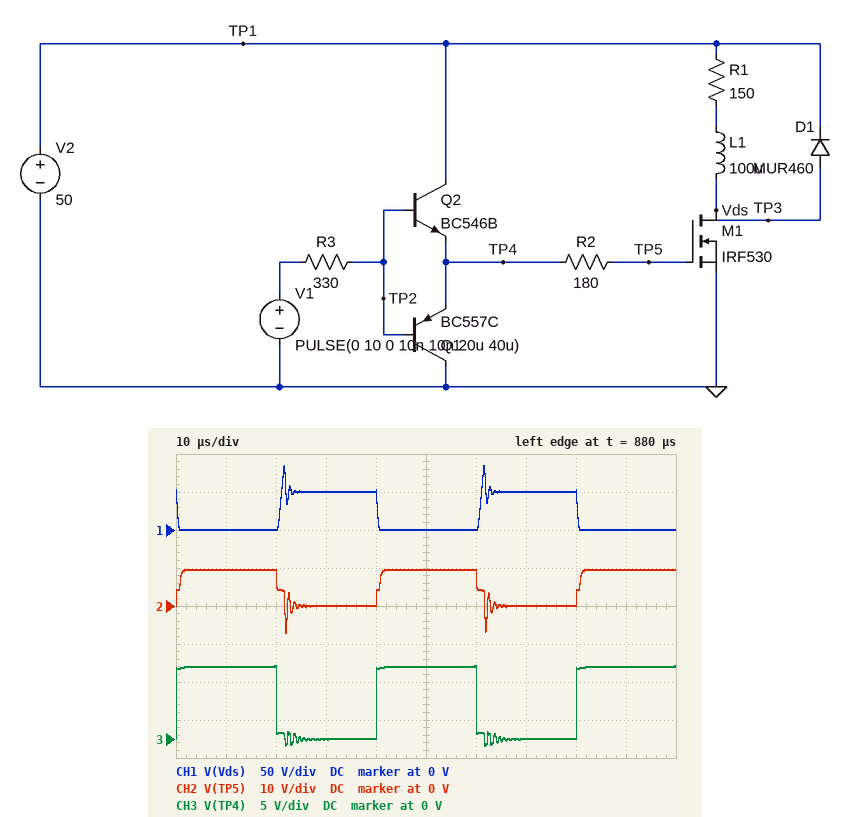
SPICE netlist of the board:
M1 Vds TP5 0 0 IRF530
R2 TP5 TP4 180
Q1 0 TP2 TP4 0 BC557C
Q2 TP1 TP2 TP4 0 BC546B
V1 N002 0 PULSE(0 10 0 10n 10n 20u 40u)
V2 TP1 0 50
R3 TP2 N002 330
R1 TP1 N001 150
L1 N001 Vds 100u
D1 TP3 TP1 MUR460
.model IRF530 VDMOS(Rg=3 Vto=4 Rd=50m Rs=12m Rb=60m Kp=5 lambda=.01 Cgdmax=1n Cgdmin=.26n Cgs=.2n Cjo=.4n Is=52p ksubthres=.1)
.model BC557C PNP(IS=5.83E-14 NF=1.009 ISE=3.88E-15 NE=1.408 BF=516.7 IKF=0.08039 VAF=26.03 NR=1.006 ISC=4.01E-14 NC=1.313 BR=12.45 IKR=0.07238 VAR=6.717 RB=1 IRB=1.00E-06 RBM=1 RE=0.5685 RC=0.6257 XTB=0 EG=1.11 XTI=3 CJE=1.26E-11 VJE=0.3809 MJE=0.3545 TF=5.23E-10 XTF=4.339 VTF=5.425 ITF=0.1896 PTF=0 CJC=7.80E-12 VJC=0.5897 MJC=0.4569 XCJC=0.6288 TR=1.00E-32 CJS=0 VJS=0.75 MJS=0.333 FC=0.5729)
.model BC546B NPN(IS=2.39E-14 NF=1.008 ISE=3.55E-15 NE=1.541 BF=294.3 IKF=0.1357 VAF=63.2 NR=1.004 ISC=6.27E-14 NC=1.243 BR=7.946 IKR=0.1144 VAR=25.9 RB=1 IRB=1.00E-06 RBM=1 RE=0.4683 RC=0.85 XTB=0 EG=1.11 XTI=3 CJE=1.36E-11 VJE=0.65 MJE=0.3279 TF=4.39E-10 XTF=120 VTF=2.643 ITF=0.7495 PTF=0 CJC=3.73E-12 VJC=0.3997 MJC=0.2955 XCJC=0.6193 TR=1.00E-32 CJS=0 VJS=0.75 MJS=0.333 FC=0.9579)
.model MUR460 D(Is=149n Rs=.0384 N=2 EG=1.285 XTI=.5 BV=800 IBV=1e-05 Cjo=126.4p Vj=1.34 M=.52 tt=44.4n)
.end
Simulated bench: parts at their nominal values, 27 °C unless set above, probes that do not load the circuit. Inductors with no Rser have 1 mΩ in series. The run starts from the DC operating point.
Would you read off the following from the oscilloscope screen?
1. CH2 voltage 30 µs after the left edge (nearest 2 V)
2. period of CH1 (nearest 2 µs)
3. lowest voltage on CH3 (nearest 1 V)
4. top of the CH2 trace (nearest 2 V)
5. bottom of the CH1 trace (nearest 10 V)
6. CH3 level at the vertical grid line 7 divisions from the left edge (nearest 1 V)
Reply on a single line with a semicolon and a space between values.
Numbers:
0 V; 40 µs; -1 V; 10 V; 0 V; 0 V
